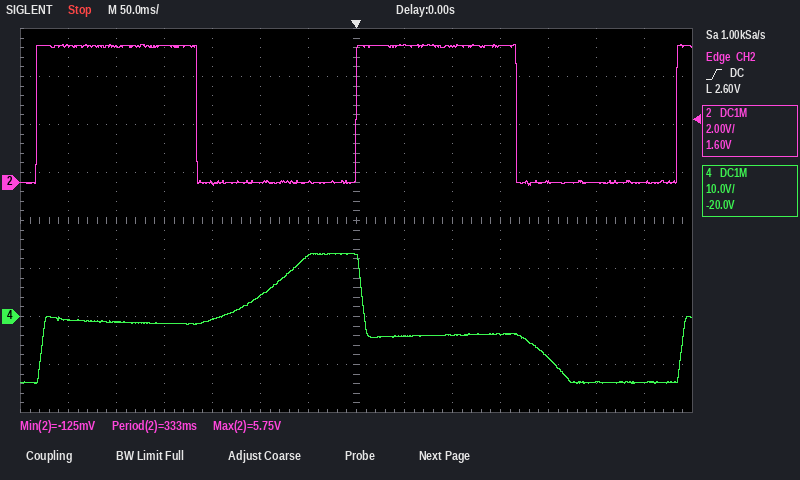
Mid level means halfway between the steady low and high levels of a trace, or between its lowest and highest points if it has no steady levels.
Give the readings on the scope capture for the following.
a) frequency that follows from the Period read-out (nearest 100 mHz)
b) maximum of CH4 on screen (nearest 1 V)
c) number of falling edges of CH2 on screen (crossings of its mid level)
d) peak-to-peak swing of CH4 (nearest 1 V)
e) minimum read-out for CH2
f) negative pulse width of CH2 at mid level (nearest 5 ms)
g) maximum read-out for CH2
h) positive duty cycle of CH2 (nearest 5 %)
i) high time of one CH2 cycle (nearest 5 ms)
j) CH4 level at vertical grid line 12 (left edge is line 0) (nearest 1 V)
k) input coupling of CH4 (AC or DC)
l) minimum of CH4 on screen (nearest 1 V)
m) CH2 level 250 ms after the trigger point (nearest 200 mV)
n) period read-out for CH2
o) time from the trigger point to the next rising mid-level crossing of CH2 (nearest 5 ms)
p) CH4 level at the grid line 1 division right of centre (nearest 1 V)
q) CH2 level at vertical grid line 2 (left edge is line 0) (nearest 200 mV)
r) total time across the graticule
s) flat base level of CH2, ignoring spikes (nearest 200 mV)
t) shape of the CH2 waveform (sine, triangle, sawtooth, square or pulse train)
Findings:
3.0 Hz
13 V
2
27 V
-125 mV
165 ms
5.75 V
50 %
165 ms
-14 V
DC
-14 V
0.0 V
333 ms
335 ms
-4 V
5.6 V
700 ms
0.0 V
square
